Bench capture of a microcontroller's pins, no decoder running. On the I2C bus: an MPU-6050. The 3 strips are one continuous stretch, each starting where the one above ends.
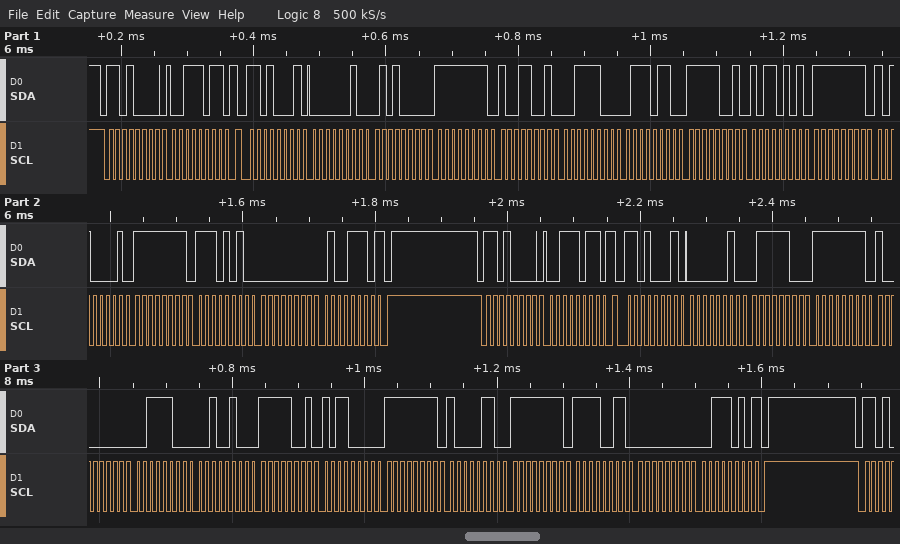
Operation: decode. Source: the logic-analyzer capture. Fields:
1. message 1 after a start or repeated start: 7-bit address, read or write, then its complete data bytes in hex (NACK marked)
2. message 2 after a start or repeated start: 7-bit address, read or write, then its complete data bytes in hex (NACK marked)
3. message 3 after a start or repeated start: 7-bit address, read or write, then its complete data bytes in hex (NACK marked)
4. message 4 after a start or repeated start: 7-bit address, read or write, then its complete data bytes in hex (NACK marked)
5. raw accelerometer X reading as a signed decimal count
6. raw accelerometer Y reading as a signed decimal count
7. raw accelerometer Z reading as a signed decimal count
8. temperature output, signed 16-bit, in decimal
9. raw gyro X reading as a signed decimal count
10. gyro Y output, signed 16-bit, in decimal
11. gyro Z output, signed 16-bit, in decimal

0x68 write: 3B
0x68 read: 02 50 FF 99 3C 76 F9 B5 FF A1 FF EA 00 4E NACK
0x68 write: 3B
0x68 read: 02 7C FF 80 3C 24 F9 B0 FF 86 FF F3 00 3A NACK
592
-103
15478
-1611
-95
-22
78
